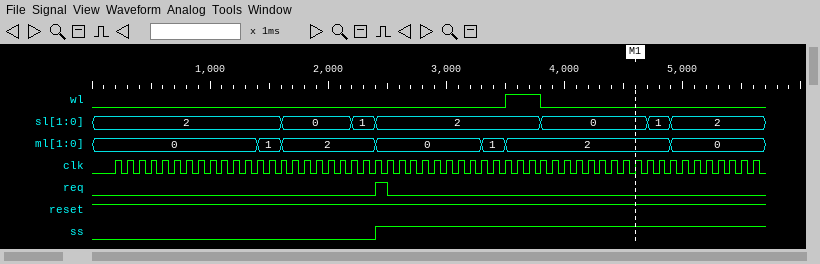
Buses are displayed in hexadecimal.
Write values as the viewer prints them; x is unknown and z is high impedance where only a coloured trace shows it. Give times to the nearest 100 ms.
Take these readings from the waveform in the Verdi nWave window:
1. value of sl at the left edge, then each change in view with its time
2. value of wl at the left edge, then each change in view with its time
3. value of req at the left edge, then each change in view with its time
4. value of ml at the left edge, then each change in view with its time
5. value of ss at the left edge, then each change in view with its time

2, 0 at 1600 ms, 1 at 2200 ms, 2 at 2400 ms, 0 at 3800 ms, 1 at 4700 ms, 2 at 4900 ms
0, 1 at 3500 ms, 0 at 3800 ms
0, 1 at 2400 ms, 0 at 2500 ms
0, 1 at 1400 ms, 2 at 1600 ms, 0 at 2400 ms, 1 at 3300 ms, 2 at 3500 ms, 0 at 4900 ms
0, 1 at 2400 ms
